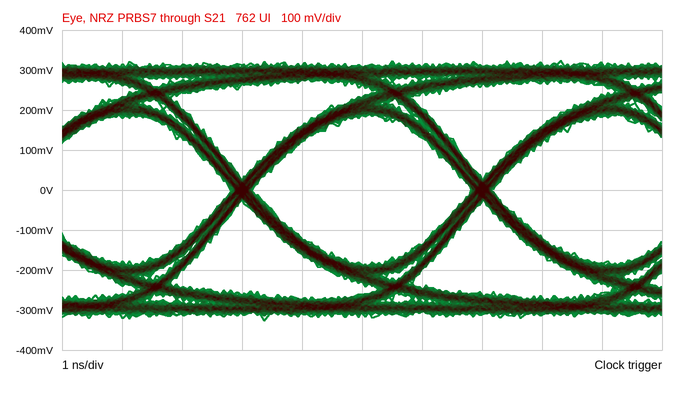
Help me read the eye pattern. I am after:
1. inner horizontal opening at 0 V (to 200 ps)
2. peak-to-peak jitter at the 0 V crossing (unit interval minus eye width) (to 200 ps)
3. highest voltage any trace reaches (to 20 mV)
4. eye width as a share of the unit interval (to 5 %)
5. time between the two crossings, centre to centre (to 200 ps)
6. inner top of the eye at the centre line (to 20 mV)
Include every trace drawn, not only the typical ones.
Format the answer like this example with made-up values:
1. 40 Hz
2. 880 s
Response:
1. 3.6 ns
2. 400 ps
3. 320 mV
4. 90 %
5. 4.0 ns
6. 180 mV
